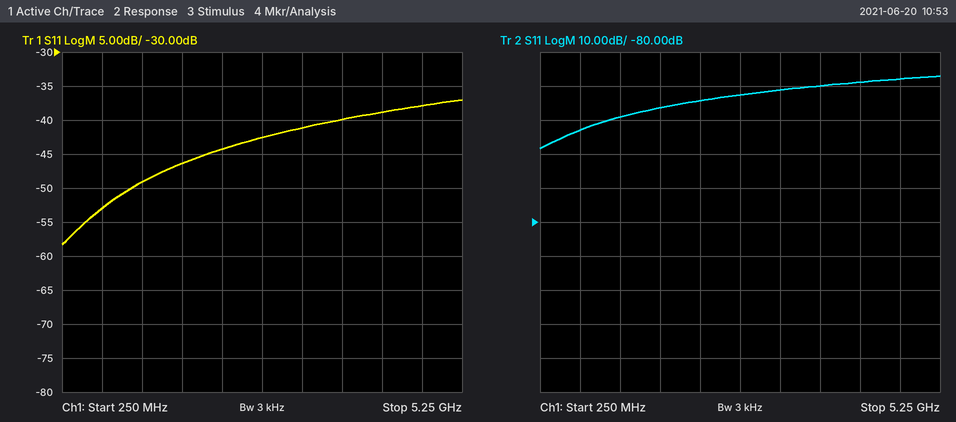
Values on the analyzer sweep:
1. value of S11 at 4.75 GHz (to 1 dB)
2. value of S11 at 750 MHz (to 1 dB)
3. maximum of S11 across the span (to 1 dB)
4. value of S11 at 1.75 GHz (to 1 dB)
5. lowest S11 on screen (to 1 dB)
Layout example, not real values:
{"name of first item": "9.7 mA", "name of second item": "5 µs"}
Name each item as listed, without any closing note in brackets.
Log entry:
{"value of S11 at 4.75 GHz": "-38 dB", "value of S11 at 750 MHz": "-53 dB", "maximum of S11 across the span": "-37 dB", "value of S11 at 1.75 GHz": "-46 dB", "lowest S11 on screen": "-58 dB"}
